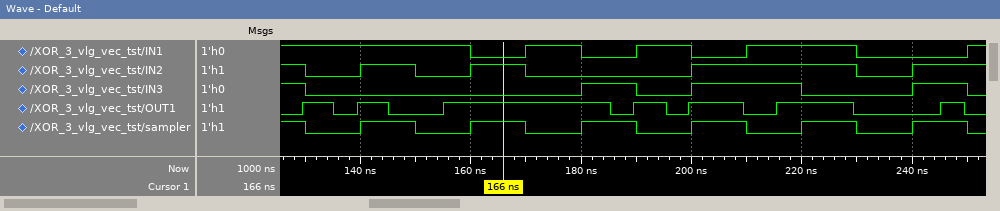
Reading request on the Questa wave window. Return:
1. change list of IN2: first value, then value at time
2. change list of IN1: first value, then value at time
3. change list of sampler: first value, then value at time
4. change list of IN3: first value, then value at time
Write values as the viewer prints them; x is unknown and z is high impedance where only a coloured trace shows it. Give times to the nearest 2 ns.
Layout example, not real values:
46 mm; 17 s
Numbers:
1, 0 at 130 ns, 1 at 140 ns, 0 at 150 ns, 1 at 160 ns, 0 at 170 ns, 1 at 200 ns, 0 at 230 ns, 1 at 240 ns; 1, 0 at 160 ns, 1 at 170 ns, 0 at 180 ns, 1 at 190 ns, 0 at 200 ns, 1 at 210 ns, 0 at 230 ns, 1 at 250 ns; 1, 0 at 130 ns, 1 at 140 ns, 0 at 150 ns, 1 at 160 ns, 0 at 170 ns, 1 at 180 ns, 0 at 190 ns, 1 at 200 ns, 0 at 210 ns, 1 at 220 ns, 0 at 230 ns, 1 at 240 ns, 0 at 250 ns; 1, 0 at 130 ns, 1 at 180 ns, 0 at 190 ns, 1 at 200 ns, 0 at 220 ns, 1 at 240 ns, 0 at 250 ns
